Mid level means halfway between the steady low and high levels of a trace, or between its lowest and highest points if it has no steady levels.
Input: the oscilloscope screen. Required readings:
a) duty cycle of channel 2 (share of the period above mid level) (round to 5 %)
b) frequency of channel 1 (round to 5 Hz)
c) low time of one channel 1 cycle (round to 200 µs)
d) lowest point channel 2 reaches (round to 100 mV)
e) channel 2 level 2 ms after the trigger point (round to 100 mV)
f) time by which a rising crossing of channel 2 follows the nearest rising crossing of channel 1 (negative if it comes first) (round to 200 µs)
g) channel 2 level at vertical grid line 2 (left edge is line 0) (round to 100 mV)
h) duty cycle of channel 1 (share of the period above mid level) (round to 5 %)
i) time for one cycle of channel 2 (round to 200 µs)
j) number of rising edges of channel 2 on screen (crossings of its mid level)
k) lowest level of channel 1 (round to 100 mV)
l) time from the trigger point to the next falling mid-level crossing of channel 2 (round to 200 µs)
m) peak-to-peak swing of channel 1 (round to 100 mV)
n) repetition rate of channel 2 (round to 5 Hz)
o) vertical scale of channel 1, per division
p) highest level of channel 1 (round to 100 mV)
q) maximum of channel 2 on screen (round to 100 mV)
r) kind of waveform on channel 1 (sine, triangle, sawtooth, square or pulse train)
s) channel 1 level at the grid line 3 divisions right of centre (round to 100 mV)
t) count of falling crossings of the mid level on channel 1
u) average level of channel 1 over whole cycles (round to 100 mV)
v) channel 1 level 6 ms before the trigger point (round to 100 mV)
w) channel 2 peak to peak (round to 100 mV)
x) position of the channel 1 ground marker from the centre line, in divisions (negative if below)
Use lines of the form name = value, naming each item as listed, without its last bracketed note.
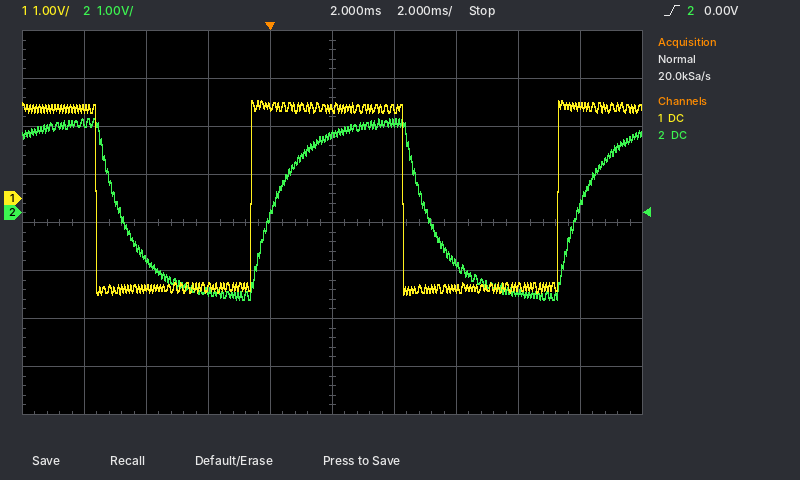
duty cycle of channel 2 (share of the period above mid level) = 50 %
frequency of channel 1 = 100 Hz
low time of one channel 1 cycle = 5.0 ms
lowest point channel 2 reaches = -1.8 V
channel 2 level 2 ms after the trigger point = 1.6 V
time by which a rising crossing of channel 2 follows the nearest rising crossing of channel 1 (negative if it comes first) = +600 µs
channel 2 level at vertical grid line 2 (left edge is line 0) = -1.0 V
duty cycle of channel 1 (share of the period above mid level) = 50 %
time for one cycle of channel 2 = 9.8 ms
number of rising edges of channel 2 on screen = 2
lowest level of channel 1 = -2.0 V
time from the trigger point to the next falling mid-level crossing of channel 2 = 5.0 ms
peak-to-peak swing of channel 1 = 4.0 V
repetition rate of channel 2 = 100 Hz
vertical scale of channel 1, per division = 1 V
highest level of channel 1 = 2.0 V
maximum of channel 2 on screen = 2.0 V
kind of waveform on channel 1 = square
channel 1 level at the grid line 3 divisions right of centre = -1.8 V
count of falling crossings of the mid level on channel 1 = 2
average level of channel 1 over whole cycles = 0.0 V
channel 1 level 6 ms before the trigger point = 1.9 V
channel 2 peak to peak = 3.8 V
position of the channel 1 ground marker from the centre line, in divisions = +0.5 div
